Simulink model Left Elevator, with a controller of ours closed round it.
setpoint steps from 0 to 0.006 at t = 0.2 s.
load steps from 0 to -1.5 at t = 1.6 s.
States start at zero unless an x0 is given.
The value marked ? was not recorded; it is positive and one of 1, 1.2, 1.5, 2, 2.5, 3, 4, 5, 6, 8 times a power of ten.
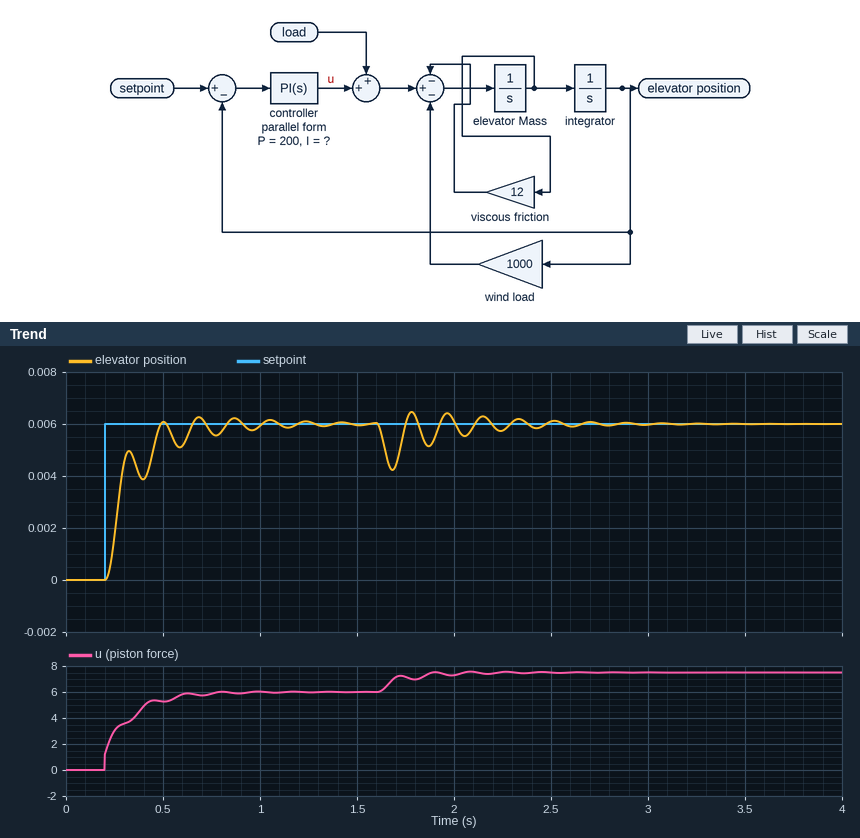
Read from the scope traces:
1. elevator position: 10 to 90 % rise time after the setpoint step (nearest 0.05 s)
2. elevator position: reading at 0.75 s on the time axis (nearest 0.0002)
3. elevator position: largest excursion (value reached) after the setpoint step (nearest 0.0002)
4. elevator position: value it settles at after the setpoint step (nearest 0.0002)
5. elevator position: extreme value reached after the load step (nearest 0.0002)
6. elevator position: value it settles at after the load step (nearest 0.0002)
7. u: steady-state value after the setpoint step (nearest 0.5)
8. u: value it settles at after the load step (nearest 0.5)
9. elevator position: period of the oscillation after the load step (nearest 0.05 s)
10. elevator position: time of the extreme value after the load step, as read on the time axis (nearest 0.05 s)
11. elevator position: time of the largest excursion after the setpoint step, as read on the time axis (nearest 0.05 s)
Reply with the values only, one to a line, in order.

0.25 s
0.0056
0.0062
0.0060
0.0042
0.0060
6.0
7.5
0.20 s
1.70 s
0.70 s
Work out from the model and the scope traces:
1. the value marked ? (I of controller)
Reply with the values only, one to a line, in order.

8000
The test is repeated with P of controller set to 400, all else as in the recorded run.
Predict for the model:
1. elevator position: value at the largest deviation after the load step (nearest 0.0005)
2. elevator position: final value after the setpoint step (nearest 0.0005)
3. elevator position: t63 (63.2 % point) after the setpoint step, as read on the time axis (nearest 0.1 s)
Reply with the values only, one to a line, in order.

0.0045
0.0060
0.3 s
